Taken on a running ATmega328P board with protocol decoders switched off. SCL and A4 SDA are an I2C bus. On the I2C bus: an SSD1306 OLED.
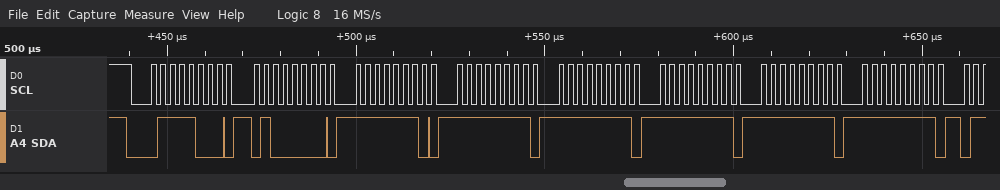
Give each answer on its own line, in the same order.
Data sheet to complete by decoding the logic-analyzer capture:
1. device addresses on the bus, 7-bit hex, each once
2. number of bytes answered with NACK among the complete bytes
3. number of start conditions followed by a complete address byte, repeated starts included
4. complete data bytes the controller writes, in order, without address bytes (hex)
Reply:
0x3C
0
1
40 FE FF FF FF FF FF
